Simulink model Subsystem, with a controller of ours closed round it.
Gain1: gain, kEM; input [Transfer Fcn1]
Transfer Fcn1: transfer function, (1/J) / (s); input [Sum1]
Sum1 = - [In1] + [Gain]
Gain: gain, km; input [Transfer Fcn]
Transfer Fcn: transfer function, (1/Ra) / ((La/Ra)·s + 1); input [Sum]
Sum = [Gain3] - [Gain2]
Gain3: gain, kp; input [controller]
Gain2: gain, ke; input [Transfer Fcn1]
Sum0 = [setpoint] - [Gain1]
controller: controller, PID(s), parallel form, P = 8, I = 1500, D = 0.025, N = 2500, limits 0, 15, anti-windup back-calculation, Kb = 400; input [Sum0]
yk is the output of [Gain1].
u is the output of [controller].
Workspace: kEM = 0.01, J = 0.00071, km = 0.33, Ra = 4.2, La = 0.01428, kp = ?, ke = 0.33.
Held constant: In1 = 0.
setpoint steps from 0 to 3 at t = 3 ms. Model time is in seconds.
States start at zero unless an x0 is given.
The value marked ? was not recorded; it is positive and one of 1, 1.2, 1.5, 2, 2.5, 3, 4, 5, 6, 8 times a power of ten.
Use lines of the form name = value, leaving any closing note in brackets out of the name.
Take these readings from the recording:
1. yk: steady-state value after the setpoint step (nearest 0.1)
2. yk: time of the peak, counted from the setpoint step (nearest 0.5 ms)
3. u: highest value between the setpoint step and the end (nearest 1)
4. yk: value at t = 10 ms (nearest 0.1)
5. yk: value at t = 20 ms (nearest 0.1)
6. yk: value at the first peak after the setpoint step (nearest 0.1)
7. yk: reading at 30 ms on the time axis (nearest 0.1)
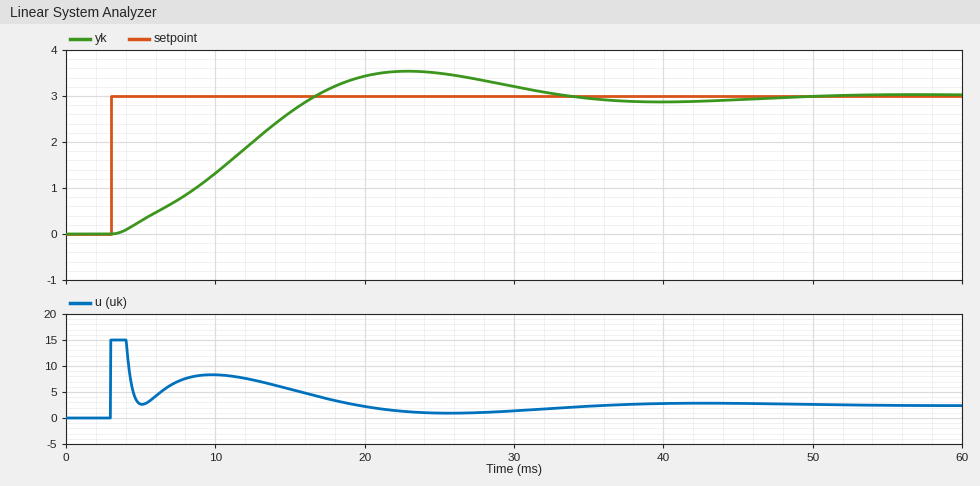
yk: steady-state value after the setpoint step = 3.0
yk: time of the peak, counted from the setpoint step = 20.0 ms
u: highest value between the setpoint step and the end = 15
yk: value at t = 10 ms = 1.3
yk: value at t = 20 ms = 3.4
yk: value at the first peak after the setpoint step = 3.5
yk: reading at 30 ms on the time axis = 3.2
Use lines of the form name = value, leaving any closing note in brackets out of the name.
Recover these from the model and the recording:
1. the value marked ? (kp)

the value marked ? = 40
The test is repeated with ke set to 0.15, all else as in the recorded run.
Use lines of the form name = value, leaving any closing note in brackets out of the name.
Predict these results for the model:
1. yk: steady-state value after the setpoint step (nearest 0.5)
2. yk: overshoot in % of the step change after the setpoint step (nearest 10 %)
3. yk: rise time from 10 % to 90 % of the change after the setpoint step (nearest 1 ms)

yk: steady-state value after the setpoint step = 3.0
yk: overshoot in % of the step change after the setpoint step = 20 %
yk: rise time from 10 % to 90 % of the change after the setpoint step = 10 ms
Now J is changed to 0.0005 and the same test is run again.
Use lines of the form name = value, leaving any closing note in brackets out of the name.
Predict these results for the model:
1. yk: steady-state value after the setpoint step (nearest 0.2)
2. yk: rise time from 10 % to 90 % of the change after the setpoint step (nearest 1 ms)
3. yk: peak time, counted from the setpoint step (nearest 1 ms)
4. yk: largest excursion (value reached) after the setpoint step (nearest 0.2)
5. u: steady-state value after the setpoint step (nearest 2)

yk: steady-state value after the setpoint step = 3.0
yk: rise time from 10 % to 90 % of the change after the setpoint step = 10 ms
yk: peak time, counted from the setpoint step = 19 ms
yk: largest excursion (value reached) after the setpoint step = 3.4
u: steady-state value after the setpoint step = 2
